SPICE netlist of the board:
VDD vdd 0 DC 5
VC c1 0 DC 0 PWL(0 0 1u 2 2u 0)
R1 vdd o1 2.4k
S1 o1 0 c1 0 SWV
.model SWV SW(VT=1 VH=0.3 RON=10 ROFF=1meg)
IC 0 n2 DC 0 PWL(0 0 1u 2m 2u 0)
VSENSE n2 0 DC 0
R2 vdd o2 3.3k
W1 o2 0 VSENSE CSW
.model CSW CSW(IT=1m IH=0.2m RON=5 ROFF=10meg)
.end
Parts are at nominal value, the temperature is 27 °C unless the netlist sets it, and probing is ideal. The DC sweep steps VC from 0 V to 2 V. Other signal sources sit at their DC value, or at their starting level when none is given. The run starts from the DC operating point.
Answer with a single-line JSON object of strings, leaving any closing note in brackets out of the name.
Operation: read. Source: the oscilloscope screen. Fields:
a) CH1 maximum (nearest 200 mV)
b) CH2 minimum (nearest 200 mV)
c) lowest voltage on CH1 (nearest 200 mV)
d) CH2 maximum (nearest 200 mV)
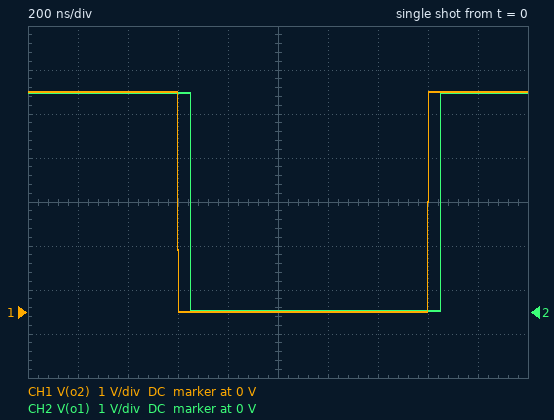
{"CH1 maximum": "5.0 V", "CH2 minimum": "0 V", "lowest voltage on CH1": "0 V", "CH2 maximum": "5.0 V"}
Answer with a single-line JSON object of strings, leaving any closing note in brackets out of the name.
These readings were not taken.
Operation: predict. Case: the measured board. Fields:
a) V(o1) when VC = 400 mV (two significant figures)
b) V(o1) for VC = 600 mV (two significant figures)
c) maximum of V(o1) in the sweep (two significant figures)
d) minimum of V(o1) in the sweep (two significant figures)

{"V(o1) when VC = 400 mV": "5.0 V", "V(o1) for VC = 600 mV": "5.0 V", "maximum of V(o1) in the sweep": "5.0 V", "minimum of V(o1) in the sweep": "21 mV"}
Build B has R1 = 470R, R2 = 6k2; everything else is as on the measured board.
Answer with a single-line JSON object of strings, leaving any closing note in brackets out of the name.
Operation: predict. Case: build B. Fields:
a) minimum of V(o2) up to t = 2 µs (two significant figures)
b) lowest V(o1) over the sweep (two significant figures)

{"minimum of V(o2) up to t = 2 µs": "4.0 mV", "lowest V(o1) over the sweep": "100 mV"}
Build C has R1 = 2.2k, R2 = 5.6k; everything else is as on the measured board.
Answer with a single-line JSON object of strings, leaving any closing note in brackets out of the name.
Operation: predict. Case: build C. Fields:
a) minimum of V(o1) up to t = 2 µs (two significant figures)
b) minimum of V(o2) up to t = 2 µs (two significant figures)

{"minimum of V(o1) up to t = 2 µs": "23 mV", "minimum of V(o2) up to t = 2 µs": "4.5 mV"}
